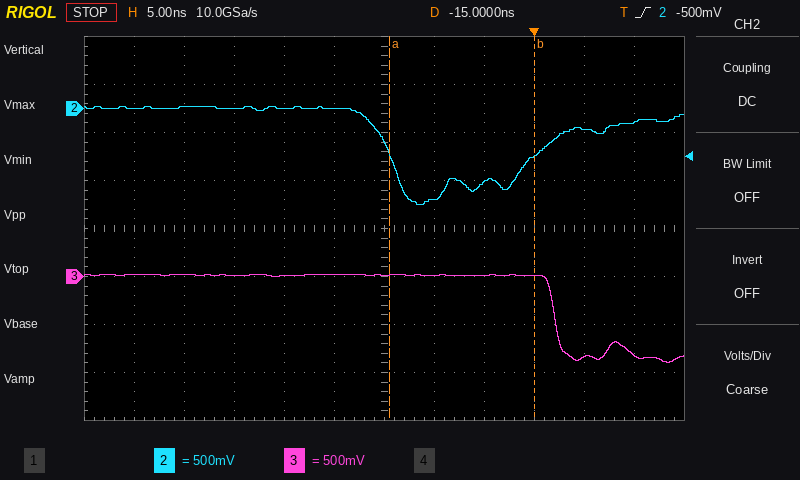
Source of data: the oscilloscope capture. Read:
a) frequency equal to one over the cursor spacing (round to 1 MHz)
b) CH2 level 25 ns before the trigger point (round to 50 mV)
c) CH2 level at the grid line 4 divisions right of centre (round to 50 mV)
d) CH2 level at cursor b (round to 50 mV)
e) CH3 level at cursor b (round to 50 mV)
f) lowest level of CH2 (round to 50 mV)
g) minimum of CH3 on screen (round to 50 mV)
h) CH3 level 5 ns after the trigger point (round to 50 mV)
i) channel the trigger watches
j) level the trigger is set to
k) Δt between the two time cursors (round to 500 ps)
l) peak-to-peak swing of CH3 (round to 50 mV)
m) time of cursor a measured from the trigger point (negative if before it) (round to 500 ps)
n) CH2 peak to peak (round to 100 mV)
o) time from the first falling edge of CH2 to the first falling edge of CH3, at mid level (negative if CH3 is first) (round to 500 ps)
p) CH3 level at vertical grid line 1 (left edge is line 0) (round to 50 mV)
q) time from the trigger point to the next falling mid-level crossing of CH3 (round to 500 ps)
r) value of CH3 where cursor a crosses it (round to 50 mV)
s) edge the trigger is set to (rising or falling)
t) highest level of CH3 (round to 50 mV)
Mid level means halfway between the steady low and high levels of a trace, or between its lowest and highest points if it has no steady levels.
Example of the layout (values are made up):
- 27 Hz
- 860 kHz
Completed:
- 69 MHz
- 0 mV
- -200 mV
- -500 mV
- 0 mV
- -1.00 V
- -900 mV
- -850 mV
- CH2
- -500 mV
- 14.5 ns
- 900 mV
- -14.5 ns
- 1.00 V
- +16.5 ns
- 0 mV
- 2.0 ns
- 0 mV
- rising
- 0 mV
